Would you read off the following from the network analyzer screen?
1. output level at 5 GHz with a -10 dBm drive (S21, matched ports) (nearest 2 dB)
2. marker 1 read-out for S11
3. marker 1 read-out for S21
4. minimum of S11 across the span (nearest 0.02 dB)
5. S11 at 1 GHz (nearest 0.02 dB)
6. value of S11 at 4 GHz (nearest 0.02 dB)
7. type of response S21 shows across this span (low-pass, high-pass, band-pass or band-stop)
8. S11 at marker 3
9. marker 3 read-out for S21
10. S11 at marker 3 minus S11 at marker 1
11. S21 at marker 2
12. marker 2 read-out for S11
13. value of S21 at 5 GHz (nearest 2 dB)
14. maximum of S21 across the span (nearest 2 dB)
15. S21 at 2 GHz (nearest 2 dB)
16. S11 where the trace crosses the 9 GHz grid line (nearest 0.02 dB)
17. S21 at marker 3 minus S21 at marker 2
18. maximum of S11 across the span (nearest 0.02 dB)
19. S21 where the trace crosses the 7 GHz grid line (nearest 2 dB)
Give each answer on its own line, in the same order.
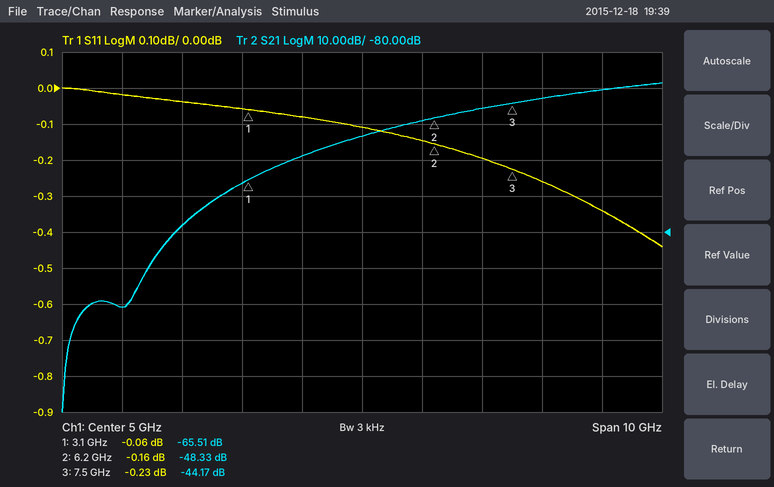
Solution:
-64 dBm
-0.06 dB
-65.51 dB
-0.44 dB
-0.02 dB
-0.08 dB
high-pass
-0.23 dB
-44.17 dB
-0.17 dB
-48.33 dB
-0.16 dB
-54 dB
-38 dB
-78 dB
-0.34 dB
4.16 dB
0.00 dB
-46 dB
